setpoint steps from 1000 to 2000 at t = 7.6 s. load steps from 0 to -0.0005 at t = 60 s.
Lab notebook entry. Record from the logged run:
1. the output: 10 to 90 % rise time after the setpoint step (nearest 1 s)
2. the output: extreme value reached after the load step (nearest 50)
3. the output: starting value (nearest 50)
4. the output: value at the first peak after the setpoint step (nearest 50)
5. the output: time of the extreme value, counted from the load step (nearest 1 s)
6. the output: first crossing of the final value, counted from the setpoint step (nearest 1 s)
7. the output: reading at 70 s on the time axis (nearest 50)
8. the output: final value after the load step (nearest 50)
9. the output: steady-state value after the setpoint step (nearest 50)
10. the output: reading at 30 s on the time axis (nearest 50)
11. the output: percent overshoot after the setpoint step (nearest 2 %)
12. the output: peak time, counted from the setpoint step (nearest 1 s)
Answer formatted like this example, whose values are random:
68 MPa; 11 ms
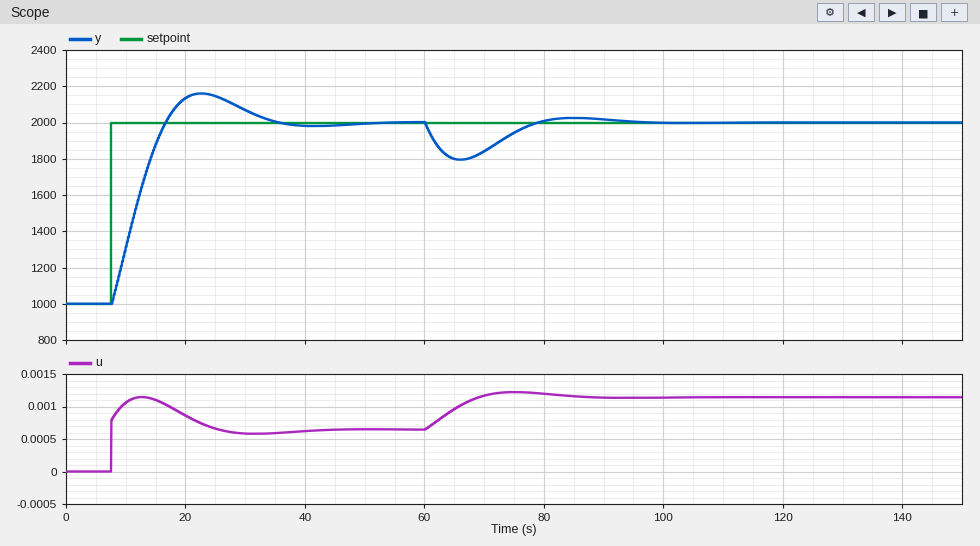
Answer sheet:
7 s; 1800; 1000; 2150; 6 s; 9 s; 1850; 2000; 2000; 2050; 16 %; 15 s
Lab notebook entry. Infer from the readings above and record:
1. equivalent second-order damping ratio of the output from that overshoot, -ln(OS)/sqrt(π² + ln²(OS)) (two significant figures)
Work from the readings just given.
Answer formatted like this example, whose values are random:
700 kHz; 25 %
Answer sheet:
0.50
